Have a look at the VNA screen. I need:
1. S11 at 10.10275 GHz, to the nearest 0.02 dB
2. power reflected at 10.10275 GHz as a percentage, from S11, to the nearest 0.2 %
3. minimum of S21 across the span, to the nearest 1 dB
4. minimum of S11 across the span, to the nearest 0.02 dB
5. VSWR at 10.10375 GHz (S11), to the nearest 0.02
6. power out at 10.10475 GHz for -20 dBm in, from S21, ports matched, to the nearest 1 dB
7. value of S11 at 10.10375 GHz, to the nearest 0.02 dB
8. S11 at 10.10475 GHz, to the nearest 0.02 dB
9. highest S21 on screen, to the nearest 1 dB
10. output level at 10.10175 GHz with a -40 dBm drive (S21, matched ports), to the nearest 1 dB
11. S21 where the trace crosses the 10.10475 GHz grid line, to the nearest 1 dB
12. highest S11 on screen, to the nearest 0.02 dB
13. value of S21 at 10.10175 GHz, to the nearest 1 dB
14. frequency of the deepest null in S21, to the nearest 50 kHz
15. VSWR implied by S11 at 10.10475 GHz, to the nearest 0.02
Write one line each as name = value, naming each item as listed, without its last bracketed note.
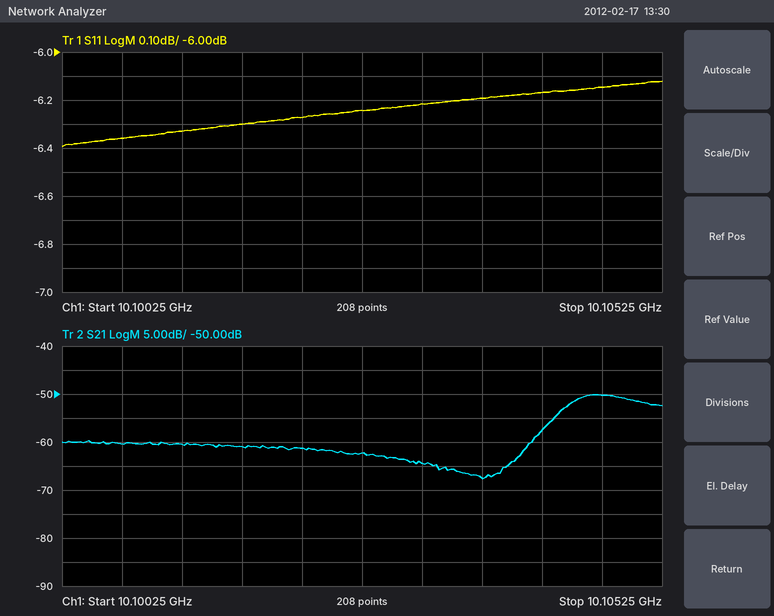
S11 at 10.10275 GHz, to the nearest 0.02 dB = -6.24 dB
power reflected at 10.10275 GHz as a percentage, from S11, to the nearest 0.2 % = 23.8 %
minimum of S21 across the span, to the nearest 1 dB = -68 dB
minimum of S11 across the span, to the nearest 0.02 dB = -6.40 dB
VSWR at 10.10375 GHz (S11), to the nearest 0.02 = 2.92
power out at 10.10475 GHz for -20 dBm in, from S21, ports matched, to the nearest 1 dB = -70 dBm
value of S11 at 10.10375 GHz, to the nearest 0.02 dB = -6.20 dB
S11 at 10.10475 GHz, to the nearest 0.02 dB = -6.14 dB
highest S21 on screen, to the nearest 1 dB = -50 dB
output level at 10.10175 GHz with a -40 dBm drive (S21, matched ports), to the nearest 1 dB = -101 dBm
S21 where the trace crosses the 10.10475 GHz grid line, to the nearest 1 dB = -50 dB
highest S11 on screen, to the nearest 0.02 dB = -6.12 dB
value of S21 at 10.10175 GHz, to the nearest 1 dB = -61 dB
frequency of the deepest null in S21, to the nearest 50 kHz = 10.10375 GHz
VSWR implied by S11 at 10.10475 GHz, to the nearest 0.02 = 2.94
